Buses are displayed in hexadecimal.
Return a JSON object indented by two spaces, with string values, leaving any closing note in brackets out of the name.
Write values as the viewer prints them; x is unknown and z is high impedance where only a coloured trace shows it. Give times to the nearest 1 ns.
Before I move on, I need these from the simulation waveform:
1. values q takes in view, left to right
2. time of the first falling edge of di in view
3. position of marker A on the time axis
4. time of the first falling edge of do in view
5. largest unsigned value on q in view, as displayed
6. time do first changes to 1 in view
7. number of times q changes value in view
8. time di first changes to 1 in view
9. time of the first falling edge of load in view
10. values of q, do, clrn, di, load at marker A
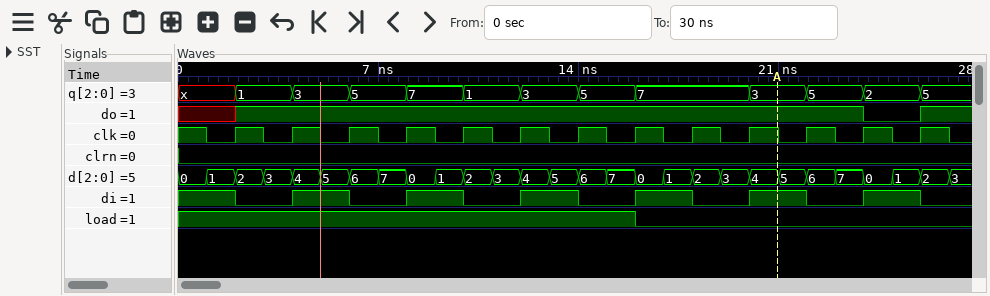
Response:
{
  "values q takes in view, left to right": "x, 1, 3, 5, 7, 1, 3, 5, 7, 3, 5, 2, 5",
  "time of the first falling edge of di in view": "2 ns",
  "position of marker A on the time axis": "21 ns",
  "time of the first falling edge of do in view": "24 ns",
  "largest unsigned value on q in view, as displayed": "7",
  "time do first changes to 1 in view": "2 ns",
  "number of times q changes value in view": "12",
  "time di first changes to 1 in view": "4 ns",
  "time of the first falling edge of load in view": "16 ns",
  "values of q, do, clrn, di, load at marker A": "q=3, do=1, clrn=0, di=1, load=0"
}
